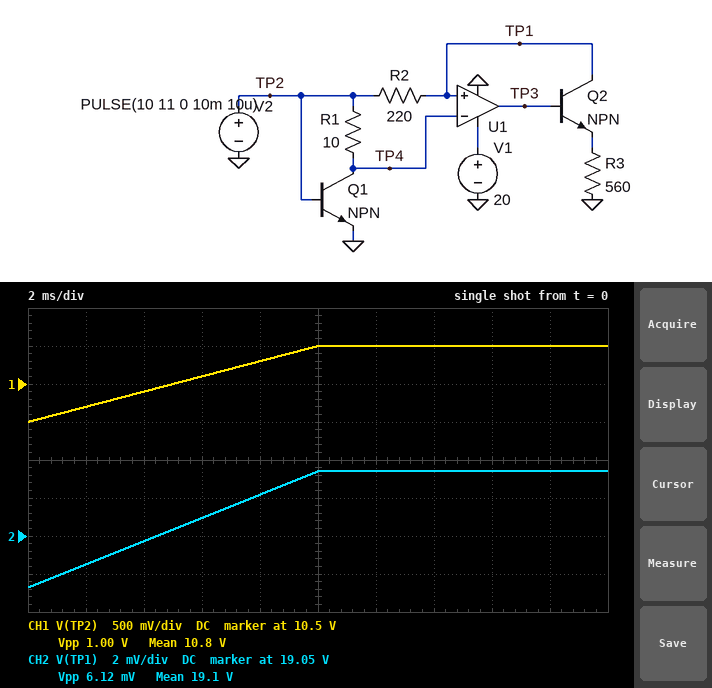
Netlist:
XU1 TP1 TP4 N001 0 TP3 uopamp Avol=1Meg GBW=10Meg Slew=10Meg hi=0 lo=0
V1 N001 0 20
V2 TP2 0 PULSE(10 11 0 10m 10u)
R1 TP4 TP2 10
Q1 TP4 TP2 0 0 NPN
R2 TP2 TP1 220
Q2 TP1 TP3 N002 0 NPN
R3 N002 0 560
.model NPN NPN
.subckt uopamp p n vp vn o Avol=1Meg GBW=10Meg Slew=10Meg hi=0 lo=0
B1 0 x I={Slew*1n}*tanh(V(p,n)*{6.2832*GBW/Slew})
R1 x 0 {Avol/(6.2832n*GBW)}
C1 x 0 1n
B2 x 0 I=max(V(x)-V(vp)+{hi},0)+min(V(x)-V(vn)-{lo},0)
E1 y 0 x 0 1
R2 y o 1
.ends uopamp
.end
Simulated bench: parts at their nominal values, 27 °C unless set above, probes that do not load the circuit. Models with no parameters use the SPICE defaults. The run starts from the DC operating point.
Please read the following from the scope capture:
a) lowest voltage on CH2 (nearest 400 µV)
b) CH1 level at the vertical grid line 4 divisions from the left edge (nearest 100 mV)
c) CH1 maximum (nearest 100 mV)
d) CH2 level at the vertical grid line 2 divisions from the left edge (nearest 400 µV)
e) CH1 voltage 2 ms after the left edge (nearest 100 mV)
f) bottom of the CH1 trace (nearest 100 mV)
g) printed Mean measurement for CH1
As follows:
19.0492 V
10.8 V
11.0 V
19.0516 V
10.2 V
10.0 V
10.8 V
